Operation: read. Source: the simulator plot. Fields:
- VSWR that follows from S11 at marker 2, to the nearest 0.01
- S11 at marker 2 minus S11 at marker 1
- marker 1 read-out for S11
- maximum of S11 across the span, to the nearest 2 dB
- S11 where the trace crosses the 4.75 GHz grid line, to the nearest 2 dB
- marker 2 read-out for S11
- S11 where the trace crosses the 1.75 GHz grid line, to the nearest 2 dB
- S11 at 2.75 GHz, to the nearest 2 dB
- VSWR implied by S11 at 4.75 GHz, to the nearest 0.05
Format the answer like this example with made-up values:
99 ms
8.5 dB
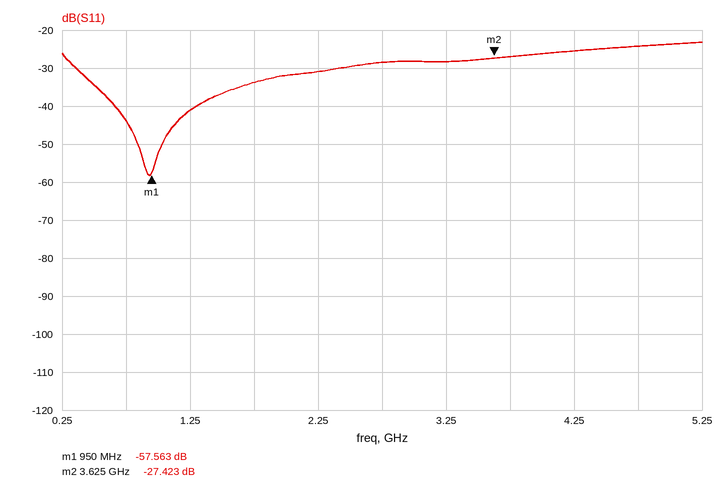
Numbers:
1.09
30.140 dB
-57.563 dB
-24 dB
-24 dB
-27.423 dB
-34 dB
-28 dB
1.15
